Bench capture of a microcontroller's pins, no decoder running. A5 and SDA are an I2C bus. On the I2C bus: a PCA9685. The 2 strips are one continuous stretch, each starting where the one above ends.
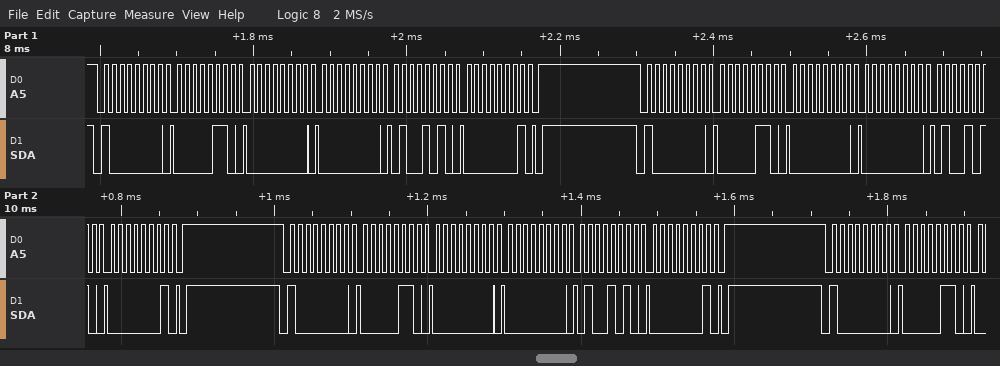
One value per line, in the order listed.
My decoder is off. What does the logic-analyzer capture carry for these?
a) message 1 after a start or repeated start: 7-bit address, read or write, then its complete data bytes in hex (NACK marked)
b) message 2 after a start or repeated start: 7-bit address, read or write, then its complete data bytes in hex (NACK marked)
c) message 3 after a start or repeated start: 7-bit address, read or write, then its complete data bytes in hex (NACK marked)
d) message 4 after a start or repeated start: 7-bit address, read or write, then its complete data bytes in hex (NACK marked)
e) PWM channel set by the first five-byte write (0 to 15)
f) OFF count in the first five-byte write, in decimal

0x40 write: 06 00 00 4A 01
0x40 write: 06 00 00 4A 01
0x40 write: 06 00 00 4A 01
0x40 write: 06
0
330
